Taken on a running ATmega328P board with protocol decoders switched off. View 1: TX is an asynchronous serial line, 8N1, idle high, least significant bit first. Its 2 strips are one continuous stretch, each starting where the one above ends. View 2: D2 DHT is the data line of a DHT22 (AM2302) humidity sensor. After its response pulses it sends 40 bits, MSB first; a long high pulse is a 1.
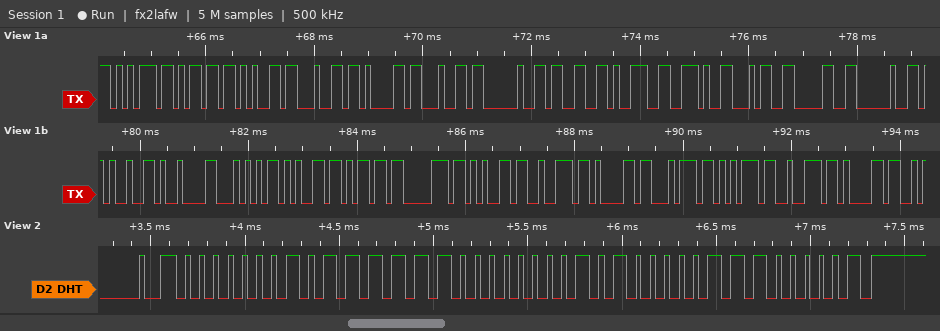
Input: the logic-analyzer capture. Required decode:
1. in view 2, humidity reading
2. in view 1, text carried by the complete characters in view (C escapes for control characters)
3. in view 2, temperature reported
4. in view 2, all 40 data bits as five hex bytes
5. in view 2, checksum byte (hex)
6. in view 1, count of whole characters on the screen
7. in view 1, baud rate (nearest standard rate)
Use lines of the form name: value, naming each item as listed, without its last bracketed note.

in view 2, humidity reading: 38.2 %
in view 1, text carried by the complete characters in view: "umedad 39.40 %\tTemperatura"
in view 2, temperature reported: 32.1 °C
in view 2, all 40 data bits as five hex bytes: 01 7E 01 41 C1
in view 2, checksum byte: 0xC1
in view 1, count of whole characters on the screen: 26
in view 1, baud rate: 9600 baud
